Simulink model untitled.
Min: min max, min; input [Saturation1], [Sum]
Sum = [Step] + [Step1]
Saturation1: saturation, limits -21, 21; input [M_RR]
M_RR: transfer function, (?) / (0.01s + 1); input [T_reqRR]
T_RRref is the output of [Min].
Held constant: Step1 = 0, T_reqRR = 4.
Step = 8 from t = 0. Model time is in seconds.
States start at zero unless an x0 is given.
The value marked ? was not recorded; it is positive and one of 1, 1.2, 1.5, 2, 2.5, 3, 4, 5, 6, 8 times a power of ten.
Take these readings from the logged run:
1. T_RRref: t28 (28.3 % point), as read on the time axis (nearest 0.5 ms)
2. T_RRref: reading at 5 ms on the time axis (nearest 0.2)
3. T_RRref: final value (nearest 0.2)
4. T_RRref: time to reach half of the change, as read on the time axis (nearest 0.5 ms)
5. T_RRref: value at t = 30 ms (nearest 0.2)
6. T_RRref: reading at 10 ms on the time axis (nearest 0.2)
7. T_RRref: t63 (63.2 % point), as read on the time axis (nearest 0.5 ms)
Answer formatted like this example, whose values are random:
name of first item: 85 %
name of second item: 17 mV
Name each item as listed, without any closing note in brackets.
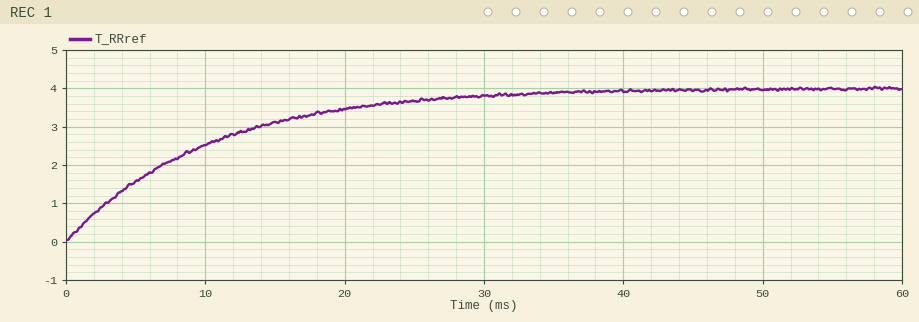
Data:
T_RRref: t28 (28.3 % point), as read on the time axis: 3.5 ms
T_RRref: reading at 5 ms on the time axis: 1.6
T_RRref: final value: 4.0
T_RRref: time to reach half of the change, as read on the time axis: 7.0 ms
T_RRref: value at t = 30 ms: 3.8
T_RRref: reading at 10 ms on the time axis: 2.6
T_RRref: t63 (63.2 % point), as read on the time axis: 10.0 ms
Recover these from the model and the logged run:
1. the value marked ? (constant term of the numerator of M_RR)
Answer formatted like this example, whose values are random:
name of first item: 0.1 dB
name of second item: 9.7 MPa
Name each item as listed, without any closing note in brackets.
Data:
the value marked ?: 1
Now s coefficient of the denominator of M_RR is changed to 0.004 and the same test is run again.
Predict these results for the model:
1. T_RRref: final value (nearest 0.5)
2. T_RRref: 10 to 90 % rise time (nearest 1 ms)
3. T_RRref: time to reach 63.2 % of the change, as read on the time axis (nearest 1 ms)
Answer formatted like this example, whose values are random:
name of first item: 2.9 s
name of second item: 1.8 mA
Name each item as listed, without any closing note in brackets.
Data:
T_RRref: final value: 4.0
T_RRref: 10 to 90 % rise time: 9 ms
T_RRref: time to reach 63.2 % of the change, as read on the time axis: 4 ms
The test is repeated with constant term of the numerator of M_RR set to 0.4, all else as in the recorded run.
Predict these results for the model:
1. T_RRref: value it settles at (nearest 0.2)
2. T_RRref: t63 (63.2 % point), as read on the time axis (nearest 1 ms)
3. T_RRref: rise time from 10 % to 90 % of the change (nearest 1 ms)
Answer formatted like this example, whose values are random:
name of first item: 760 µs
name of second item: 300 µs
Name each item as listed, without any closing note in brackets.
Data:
T_RRref: value it settles at: 1.6
T_RRref: t63 (63.2 % point), as read on the time axis: 10 ms
T_RRref: rise time from 10 % to 90 % of the change: 22 ms
